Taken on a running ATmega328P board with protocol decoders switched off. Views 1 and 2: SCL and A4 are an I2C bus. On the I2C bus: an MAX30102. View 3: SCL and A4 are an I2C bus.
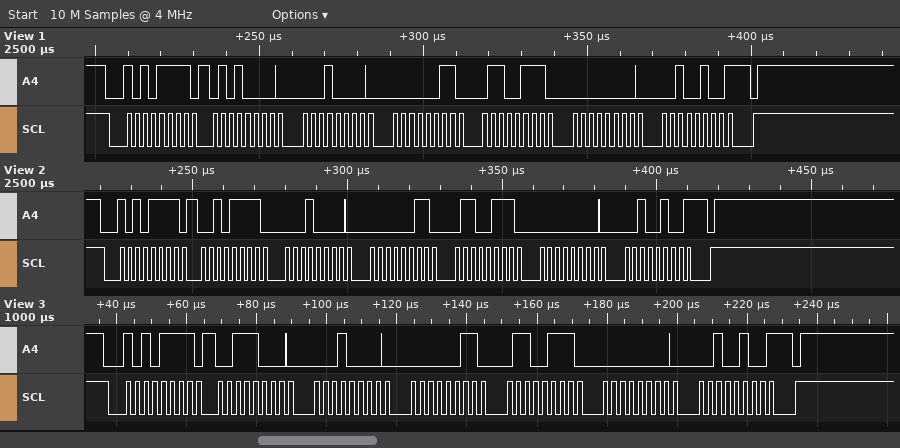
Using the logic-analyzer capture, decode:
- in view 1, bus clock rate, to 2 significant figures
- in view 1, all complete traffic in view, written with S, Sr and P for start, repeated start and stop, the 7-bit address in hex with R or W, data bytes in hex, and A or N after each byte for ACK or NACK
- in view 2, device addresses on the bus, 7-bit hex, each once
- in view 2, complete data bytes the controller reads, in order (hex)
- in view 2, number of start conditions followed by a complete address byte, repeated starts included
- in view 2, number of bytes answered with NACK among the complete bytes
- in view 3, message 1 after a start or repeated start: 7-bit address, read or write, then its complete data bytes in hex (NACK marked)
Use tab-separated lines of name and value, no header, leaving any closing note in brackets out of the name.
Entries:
in view 1, bus clock rate, to 2 significant figures	400 kHz
in view 1, all complete traffic in view, written with S, Sr and P for start, repeated start and stop, the 7-bit address in hex with R or W, data bytes in hex, and A or N after each byte for ACK or NACK	S 57R A 50 A 10 A 03 A 67 A 00 A 24 N P
in view 2, device addresses on the bus, 7-bit hex, each once	0x57
in view 2, complete data bytes the controller reads, in order	2F 10 03 67 00 24
in view 2, number of start conditions followed by a complete address byte, repeated starts included	1
in view 2, number of bytes answered with NACK among the complete bytes	1
in view 3, message 1 after a start or repeated start: 7-bit address, read or write, then its complete data bytes in hex	0x57 read: 38 10 03 67 00 24 NACK
